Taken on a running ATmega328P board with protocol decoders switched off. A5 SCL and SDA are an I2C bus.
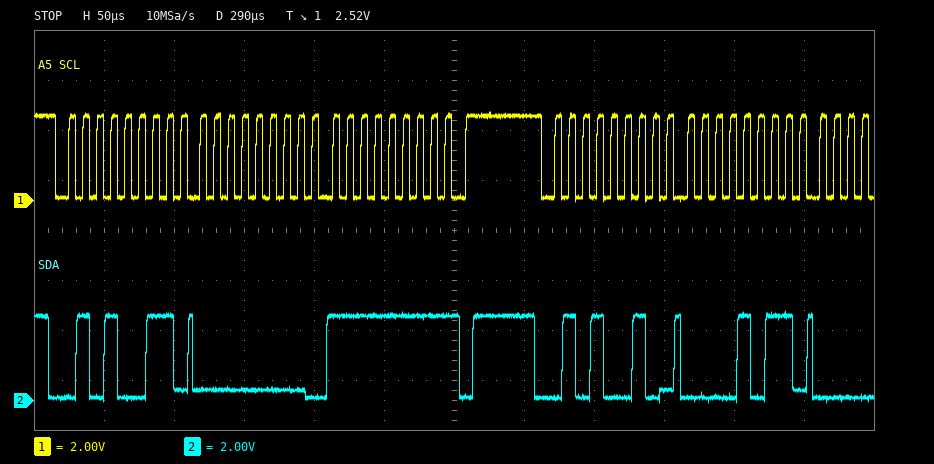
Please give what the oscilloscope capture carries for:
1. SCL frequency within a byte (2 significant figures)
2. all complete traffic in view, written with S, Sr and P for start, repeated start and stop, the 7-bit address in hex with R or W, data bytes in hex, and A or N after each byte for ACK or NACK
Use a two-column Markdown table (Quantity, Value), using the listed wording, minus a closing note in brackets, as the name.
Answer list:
| Quantity | Value |
|---|---|
| SCL frequency within a byte | 100 kHz |
| all complete traffic in view, written with S, Sr and P for start, repeated start and stop, the 7-bit address in hex with R or W, data bytes in hex, and A or N after each byte for ACK or NACK | S 29R A 00 A FF N P S 29W A 0B A |
